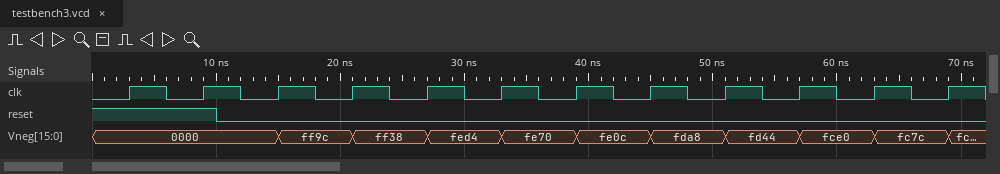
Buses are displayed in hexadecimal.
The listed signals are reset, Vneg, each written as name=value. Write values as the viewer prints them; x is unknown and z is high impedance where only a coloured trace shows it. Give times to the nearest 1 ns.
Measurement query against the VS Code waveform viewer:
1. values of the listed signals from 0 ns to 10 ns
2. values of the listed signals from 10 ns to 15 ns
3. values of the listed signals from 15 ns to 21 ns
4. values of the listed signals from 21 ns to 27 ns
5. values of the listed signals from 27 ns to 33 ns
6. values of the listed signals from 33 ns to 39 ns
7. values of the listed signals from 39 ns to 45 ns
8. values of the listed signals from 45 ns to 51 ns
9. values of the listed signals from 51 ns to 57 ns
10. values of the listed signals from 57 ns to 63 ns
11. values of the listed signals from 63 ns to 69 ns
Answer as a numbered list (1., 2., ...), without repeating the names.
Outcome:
1. reset=1, Vneg=0000
2. reset=0, Vneg=0000
3. reset=0, Vneg=ff9c
4. reset=0, Vneg=ff38
5. reset=0, Vneg=fed4
6. reset=0, Vneg=fe70
7. reset=0, Vneg=fe0c
8. reset=0, Vneg=fda8
9. reset=0, Vneg=fd44
10. reset=0, Vneg=fce0
11. reset=0, Vneg=fc7c
